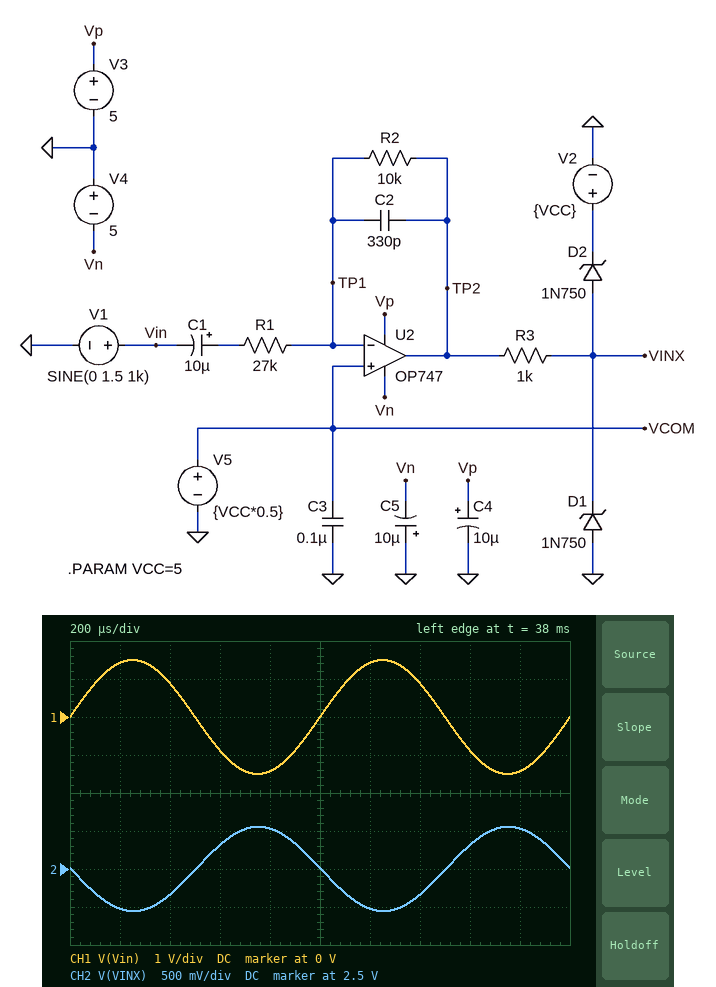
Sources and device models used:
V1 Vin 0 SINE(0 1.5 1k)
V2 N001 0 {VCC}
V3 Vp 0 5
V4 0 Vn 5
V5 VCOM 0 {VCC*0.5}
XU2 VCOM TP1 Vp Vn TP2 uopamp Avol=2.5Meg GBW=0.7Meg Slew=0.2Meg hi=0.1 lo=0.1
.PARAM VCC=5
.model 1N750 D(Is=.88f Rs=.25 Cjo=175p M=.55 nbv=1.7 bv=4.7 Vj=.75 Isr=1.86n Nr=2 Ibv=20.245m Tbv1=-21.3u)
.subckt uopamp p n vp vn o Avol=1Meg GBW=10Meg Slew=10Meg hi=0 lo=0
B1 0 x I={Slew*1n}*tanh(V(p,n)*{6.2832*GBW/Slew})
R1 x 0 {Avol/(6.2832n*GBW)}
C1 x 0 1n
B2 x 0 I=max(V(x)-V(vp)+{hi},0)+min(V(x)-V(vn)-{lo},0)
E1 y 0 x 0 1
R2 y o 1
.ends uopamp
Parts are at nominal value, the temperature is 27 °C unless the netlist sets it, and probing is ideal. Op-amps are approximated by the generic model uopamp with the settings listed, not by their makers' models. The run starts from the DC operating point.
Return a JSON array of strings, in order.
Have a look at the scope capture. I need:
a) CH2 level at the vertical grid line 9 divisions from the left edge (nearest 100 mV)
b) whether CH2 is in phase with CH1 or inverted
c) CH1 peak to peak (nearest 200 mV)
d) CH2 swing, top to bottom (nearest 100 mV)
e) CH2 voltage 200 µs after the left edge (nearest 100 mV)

["3.0 V", "inverted", "3.0 V", "1.1 V", "2.0 V"]
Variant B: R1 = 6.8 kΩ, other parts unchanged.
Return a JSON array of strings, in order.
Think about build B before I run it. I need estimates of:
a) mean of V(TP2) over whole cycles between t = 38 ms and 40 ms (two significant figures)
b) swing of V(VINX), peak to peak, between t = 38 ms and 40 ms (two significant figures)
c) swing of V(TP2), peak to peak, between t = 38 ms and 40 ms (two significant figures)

["2.5 V", "4.0 V", "4.4 V"]
